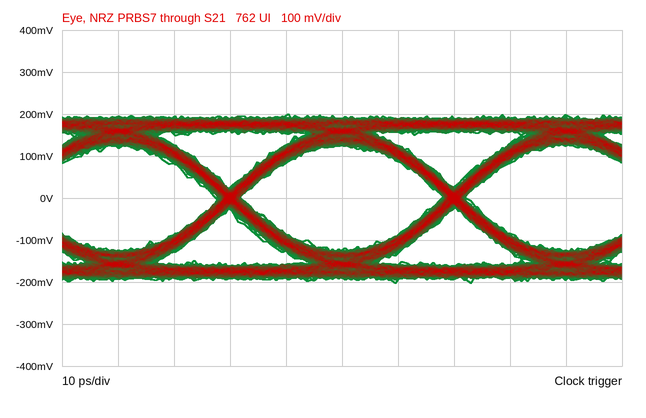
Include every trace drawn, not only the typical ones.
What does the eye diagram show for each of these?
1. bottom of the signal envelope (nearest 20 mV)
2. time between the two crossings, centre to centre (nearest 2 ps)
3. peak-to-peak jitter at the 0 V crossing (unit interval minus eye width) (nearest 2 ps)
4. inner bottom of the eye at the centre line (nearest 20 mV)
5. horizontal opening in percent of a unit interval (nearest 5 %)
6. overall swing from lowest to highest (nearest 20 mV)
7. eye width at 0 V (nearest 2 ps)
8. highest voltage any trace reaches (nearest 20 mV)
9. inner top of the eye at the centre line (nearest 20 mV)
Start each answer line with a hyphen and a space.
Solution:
- -200 mV
- 40 ps
- 4 ps
- -120 mV
- 90 %
- 400 mV
- 36 ps
- 200 mV
- 120 mV
